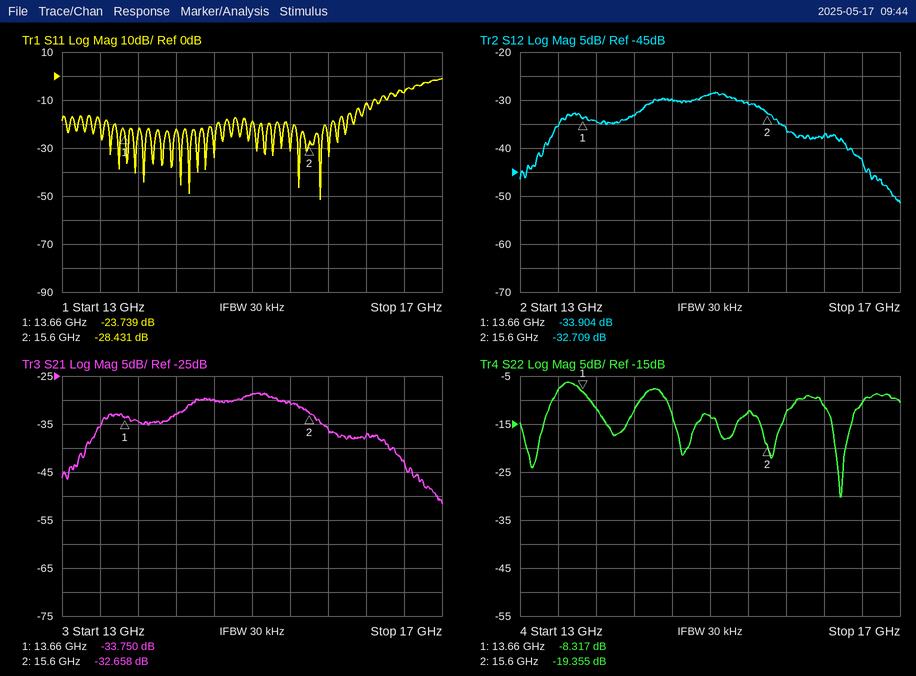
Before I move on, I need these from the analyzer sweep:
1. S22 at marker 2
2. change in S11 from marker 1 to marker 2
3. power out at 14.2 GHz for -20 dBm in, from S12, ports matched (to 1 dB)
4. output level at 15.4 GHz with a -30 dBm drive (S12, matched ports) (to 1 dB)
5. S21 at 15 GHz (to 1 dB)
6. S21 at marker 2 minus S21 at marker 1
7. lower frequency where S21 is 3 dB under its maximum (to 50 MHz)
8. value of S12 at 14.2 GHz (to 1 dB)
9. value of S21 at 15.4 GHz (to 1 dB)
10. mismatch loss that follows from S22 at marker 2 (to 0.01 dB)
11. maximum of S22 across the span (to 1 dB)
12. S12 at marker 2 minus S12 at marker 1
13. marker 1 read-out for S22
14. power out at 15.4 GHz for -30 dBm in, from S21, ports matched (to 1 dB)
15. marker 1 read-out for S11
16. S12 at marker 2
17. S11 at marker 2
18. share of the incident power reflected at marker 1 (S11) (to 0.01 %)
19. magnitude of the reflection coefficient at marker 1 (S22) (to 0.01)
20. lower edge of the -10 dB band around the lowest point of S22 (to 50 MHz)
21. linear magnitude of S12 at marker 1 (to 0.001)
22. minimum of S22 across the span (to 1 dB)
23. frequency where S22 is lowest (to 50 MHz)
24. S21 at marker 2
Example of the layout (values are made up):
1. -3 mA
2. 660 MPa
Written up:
1. -19.355 dB
2. -4.692 dB
3. -53 dBm
4. -61 dBm
5. -29 dB
6. 1.092 dB
7. 14.30 GHz
8. -33 dB
9. -31 dB
10. 0.05 dB
11. -6 dB
12. 1.195 dB
13. -8.317 dB
14. -61 dBm
15. -23.739 dB
16. -32.709 dB
17. -28.431 dB
18. 0.42 %
19. 0.38
20. 16.15 GHz
21. 0.020
22. -30 dB
23. 16.35 GHz
24. -32.658 dB
